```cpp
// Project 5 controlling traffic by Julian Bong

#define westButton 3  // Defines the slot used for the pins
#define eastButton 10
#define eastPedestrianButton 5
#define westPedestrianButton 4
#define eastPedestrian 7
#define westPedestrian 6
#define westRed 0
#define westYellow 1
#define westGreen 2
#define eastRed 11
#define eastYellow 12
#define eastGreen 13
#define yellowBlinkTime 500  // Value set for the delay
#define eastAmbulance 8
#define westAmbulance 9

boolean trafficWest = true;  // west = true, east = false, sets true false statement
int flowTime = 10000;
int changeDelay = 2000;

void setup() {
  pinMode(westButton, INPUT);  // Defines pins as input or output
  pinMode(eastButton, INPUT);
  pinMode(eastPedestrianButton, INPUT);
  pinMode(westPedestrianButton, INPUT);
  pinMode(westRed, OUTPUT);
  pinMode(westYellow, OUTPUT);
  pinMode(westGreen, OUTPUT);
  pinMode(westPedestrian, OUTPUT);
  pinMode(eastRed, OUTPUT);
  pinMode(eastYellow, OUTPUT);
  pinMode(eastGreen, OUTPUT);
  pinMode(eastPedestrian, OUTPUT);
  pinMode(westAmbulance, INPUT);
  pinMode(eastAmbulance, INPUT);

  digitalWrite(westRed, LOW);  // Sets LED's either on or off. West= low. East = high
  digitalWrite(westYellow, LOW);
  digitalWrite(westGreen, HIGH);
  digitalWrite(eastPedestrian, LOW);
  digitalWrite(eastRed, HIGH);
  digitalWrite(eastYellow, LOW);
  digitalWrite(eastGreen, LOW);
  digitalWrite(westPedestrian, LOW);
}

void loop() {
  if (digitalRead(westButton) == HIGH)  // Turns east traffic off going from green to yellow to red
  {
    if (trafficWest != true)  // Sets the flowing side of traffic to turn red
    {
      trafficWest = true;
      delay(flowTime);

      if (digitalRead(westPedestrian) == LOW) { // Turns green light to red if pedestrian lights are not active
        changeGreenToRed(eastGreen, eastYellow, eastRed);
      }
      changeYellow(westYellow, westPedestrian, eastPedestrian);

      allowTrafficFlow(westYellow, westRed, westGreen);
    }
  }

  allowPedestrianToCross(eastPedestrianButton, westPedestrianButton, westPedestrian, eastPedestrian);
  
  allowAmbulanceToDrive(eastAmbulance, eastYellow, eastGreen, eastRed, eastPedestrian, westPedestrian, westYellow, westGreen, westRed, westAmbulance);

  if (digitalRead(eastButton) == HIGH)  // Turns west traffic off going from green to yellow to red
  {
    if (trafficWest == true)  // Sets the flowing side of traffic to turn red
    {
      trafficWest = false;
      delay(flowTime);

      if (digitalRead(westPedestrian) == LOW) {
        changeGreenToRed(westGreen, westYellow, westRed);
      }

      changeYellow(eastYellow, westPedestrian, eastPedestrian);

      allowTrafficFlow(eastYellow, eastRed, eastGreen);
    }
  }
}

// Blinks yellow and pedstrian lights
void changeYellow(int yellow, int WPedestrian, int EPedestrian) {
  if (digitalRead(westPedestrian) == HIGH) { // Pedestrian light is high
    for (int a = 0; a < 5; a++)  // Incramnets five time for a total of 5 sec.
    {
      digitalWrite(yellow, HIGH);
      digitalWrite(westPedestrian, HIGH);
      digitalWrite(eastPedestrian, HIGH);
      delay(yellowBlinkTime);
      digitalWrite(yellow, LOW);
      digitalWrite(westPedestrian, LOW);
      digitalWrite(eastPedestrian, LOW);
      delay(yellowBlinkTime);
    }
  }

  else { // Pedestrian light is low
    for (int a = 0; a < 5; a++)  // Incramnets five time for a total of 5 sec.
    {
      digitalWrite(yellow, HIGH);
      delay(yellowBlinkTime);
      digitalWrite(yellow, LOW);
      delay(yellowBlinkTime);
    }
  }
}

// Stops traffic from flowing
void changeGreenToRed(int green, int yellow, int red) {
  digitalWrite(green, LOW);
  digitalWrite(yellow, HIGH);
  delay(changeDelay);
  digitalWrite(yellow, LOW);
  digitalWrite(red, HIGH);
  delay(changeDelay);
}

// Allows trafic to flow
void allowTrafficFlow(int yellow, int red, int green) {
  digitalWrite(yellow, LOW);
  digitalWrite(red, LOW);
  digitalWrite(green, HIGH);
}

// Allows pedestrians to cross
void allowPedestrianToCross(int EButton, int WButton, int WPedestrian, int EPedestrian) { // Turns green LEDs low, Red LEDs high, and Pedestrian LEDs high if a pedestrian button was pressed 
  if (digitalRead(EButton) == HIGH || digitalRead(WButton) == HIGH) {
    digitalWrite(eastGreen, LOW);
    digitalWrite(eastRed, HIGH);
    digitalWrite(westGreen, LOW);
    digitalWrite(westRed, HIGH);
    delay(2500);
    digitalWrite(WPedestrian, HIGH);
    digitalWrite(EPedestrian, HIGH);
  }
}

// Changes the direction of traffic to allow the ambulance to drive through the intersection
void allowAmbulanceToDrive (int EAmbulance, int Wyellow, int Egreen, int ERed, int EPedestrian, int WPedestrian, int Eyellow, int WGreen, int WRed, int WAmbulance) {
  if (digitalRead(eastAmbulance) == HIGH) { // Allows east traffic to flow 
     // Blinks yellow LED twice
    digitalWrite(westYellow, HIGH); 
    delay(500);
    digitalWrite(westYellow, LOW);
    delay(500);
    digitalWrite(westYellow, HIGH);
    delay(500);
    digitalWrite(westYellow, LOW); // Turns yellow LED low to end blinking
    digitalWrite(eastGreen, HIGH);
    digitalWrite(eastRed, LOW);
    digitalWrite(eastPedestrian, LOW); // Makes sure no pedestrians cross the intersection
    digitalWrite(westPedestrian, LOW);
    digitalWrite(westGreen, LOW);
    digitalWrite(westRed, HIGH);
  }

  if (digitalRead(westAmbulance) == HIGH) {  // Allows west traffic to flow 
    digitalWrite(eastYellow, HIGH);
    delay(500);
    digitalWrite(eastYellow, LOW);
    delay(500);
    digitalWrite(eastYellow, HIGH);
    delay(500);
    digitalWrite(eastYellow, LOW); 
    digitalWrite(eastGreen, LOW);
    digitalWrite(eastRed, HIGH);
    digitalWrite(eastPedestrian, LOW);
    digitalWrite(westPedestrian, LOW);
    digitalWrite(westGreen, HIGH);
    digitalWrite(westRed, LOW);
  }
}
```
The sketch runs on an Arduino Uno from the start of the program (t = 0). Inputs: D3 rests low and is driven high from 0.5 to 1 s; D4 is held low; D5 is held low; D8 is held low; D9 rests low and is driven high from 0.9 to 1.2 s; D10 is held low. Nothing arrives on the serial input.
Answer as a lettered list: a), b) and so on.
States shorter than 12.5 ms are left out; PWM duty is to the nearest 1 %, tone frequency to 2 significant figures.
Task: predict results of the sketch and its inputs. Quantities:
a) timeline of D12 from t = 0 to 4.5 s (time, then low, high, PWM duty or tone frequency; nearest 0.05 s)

a) 0 s low; 0.9 s high; 1.4 s low; 1.9 s high; 2.4 s low
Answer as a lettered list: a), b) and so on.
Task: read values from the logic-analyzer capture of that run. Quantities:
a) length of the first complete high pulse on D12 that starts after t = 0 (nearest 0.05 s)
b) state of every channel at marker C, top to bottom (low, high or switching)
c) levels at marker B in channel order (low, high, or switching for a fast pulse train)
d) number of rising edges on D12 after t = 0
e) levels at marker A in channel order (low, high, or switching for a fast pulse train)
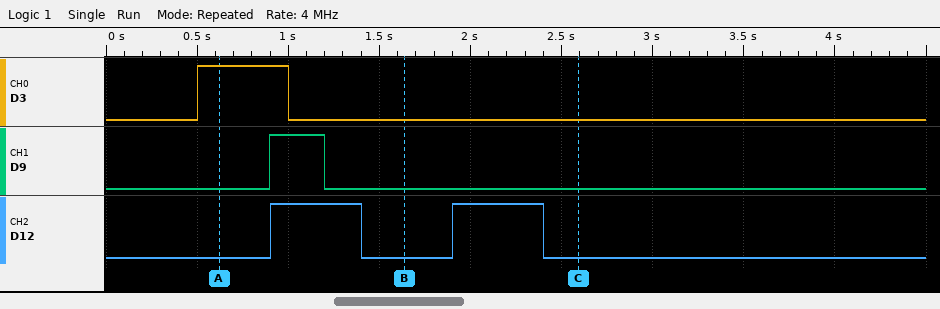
a) 0.50 s
b) D3 low, D9 low, D12 low
c) D3 low, D9 low, D12 low
d) 2
e) D3 high, D9 low, D12 low
